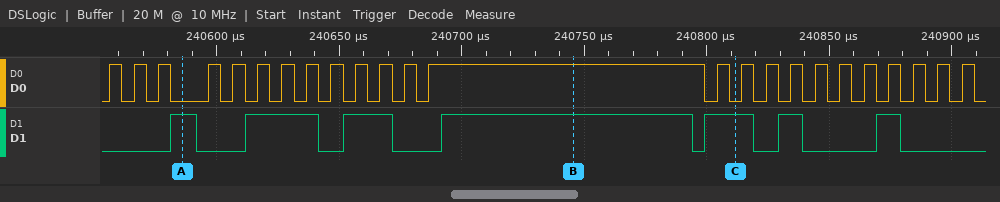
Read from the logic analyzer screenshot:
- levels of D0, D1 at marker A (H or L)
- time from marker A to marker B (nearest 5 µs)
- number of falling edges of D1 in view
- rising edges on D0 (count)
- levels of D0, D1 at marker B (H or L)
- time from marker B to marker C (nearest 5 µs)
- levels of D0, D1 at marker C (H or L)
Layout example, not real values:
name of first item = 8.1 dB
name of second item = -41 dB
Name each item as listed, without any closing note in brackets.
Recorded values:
levels of D0, D1 at marker A = D0=L, D1=H
time from marker A to marker B = 160 µs
number of falling edges of D1 in view = 7
rising edges on D0 = 24
levels of D0, D1 at marker B = D0=H, D1=H
time from marker B to marker C = 65 µs
levels of D0, D1 at marker C = D0=L, D1=H
